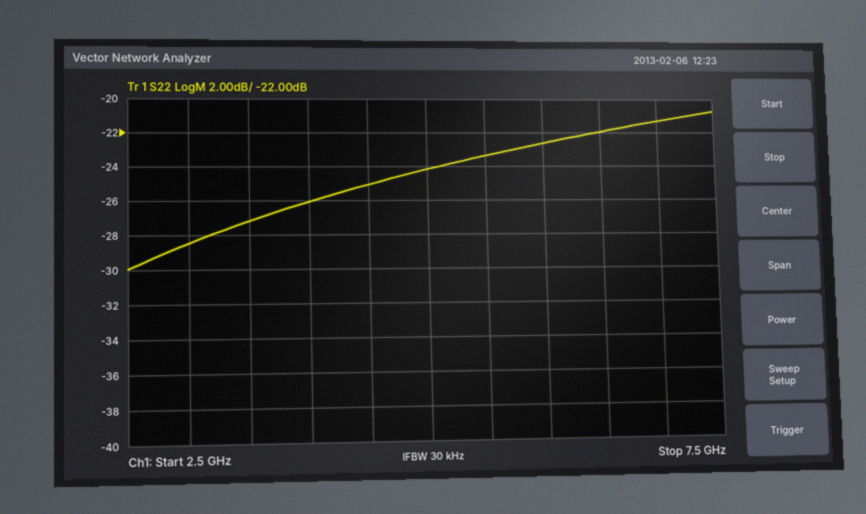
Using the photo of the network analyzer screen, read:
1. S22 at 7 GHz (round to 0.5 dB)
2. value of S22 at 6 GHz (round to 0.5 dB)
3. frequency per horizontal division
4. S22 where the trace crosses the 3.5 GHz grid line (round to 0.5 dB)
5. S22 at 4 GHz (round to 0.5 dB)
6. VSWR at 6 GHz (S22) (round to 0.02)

-21.5 dB
-22.5 dB
500 MHz
-27.0 dB
-26.0 dB
1.16
